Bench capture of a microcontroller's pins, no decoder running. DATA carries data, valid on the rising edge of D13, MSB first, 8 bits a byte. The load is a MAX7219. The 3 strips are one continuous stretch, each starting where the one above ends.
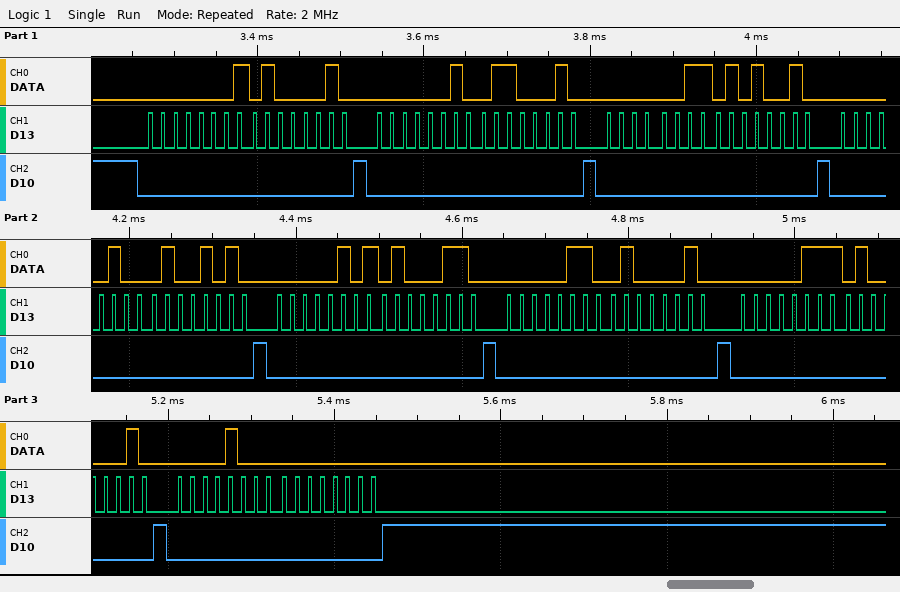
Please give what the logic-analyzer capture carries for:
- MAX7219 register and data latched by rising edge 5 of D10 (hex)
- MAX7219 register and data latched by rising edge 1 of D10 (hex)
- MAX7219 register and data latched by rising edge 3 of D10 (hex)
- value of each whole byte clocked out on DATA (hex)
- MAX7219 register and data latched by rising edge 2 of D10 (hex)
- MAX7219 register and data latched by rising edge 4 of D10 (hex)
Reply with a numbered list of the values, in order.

1. register 0x5, data 0x46
2. register 0x1, data 0x42
3. register 0x3, data 0x52
4. 01 42 02 62 03 52 04 4A 05 46 06 42 07 42 08 00
5. register 0x2, data 0x62
6. register 0x4, data 0x4A
